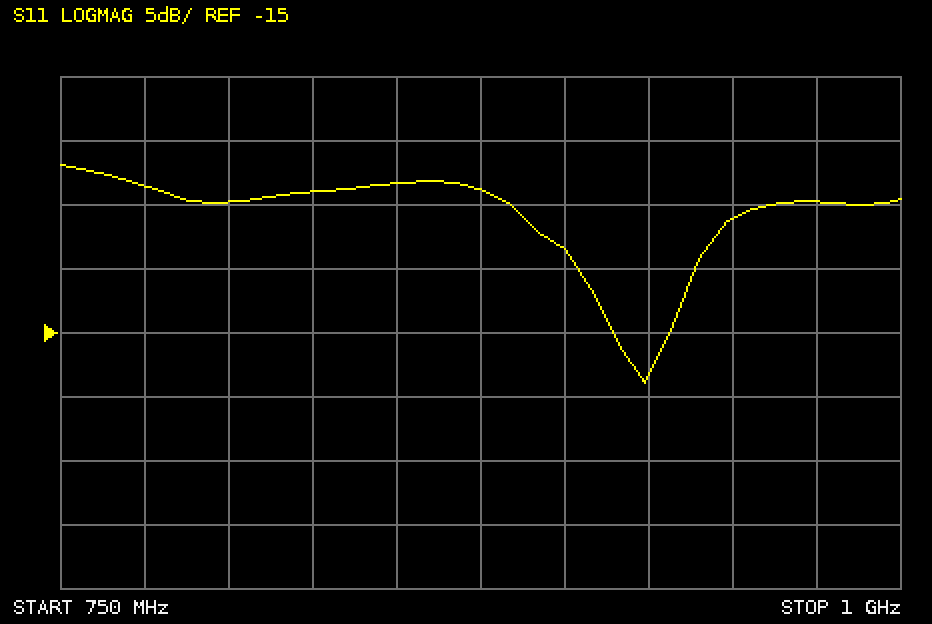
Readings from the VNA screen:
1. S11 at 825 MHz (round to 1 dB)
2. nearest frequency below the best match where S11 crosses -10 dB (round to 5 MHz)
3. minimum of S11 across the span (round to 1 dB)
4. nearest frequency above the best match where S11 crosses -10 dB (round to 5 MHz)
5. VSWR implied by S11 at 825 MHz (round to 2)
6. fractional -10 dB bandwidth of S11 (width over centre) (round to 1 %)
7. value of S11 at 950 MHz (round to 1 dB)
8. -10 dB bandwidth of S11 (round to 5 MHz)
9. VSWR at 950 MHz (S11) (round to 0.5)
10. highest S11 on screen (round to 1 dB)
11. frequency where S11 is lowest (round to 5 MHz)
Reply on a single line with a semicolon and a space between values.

-4 dB; 905 MHz; -19 dB; 940 MHz; 4; 4 %; -6 dB; 35 MHz; 3.0; -2 dB; 925 MHz
